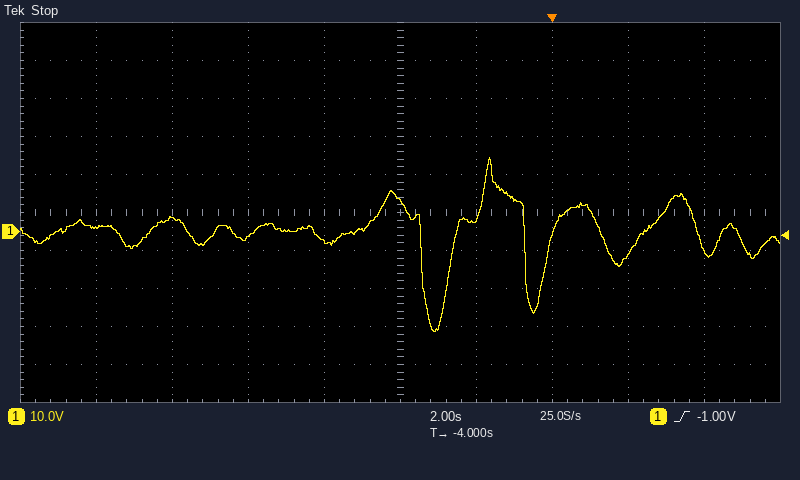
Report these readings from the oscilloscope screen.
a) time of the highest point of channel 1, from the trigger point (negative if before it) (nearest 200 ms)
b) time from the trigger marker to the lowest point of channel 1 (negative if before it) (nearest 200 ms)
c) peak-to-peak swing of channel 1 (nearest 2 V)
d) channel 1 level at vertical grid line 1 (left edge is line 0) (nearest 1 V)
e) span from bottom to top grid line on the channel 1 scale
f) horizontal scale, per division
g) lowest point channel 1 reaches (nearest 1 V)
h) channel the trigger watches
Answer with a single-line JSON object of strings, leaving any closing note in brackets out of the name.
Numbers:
{"time of the highest point of channel 1, from the trigger point (negative if before it)": "-1.6 s", "time from the trigger marker to the lowest point of channel 1 (negative if before it)": "-3.0 s", "peak-to-peak swing of channel 1": "46 V", "channel 1 level at vertical grid line 1 (left edge is line 0)": "1 V", "span from bottom to top grid line on the channel 1 scale": "100 V", "horizontal scale, per division": "2 s", "lowest point channel 1 reaches": "-26 V", "channel the trigger watches": "channel 1"}
